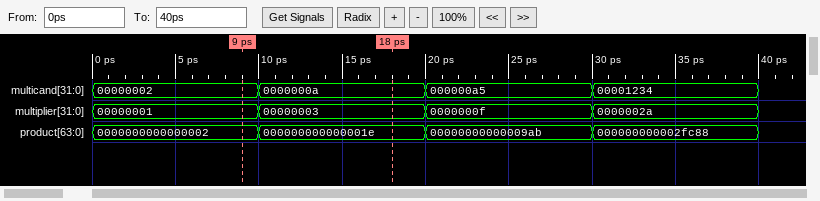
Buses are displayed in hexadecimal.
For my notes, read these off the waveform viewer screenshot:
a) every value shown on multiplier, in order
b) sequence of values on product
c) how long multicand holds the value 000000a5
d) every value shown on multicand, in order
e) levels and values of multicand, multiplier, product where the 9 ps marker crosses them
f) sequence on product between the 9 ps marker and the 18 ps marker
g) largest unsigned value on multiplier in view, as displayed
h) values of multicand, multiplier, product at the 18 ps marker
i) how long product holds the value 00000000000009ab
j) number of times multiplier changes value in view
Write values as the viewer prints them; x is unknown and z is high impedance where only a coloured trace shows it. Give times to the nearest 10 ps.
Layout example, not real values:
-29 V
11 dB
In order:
00000001, 00000003, 0000000f, 0000002a
0000000000000002, 000000000000001e, 00000000000009ab, 000000000002fc88
10 ps
00000002, 0000000a, 000000a5, 00001234
multicand=00000002, multiplier=00000001, product=0000000000000002
0000000000000002, 000000000000001e
0000002a
multicand=0000000a, multiplier=00000003, product=000000000000001e
10 ps
3
